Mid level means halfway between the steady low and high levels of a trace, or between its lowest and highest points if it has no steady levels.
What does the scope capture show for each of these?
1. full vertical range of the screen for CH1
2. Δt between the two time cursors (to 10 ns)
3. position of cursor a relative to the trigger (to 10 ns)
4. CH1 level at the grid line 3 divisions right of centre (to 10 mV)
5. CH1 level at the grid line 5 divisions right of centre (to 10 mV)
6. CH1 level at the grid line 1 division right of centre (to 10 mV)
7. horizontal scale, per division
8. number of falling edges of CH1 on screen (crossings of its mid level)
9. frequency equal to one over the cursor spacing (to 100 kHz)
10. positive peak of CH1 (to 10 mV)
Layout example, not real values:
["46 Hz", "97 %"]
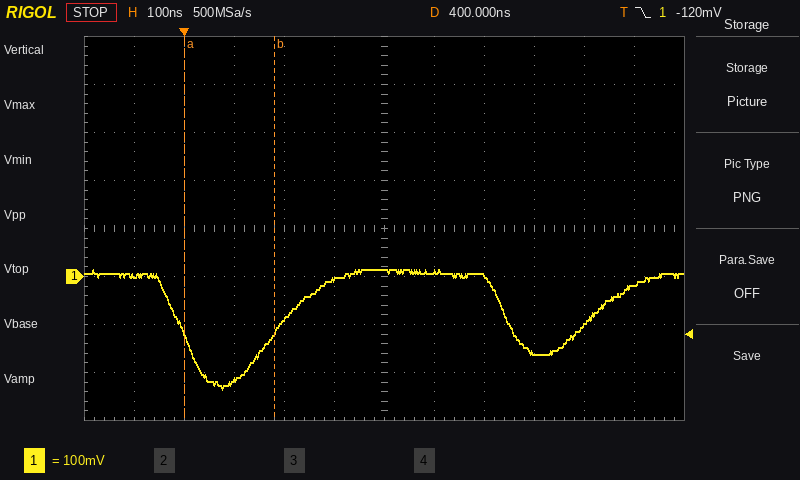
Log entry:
["800 mV", "180 ns", "0 ns", "-160 mV", "-20 mV", "10 mV", "100 ns", "2", "5.6 MHz", "10 mV"]
